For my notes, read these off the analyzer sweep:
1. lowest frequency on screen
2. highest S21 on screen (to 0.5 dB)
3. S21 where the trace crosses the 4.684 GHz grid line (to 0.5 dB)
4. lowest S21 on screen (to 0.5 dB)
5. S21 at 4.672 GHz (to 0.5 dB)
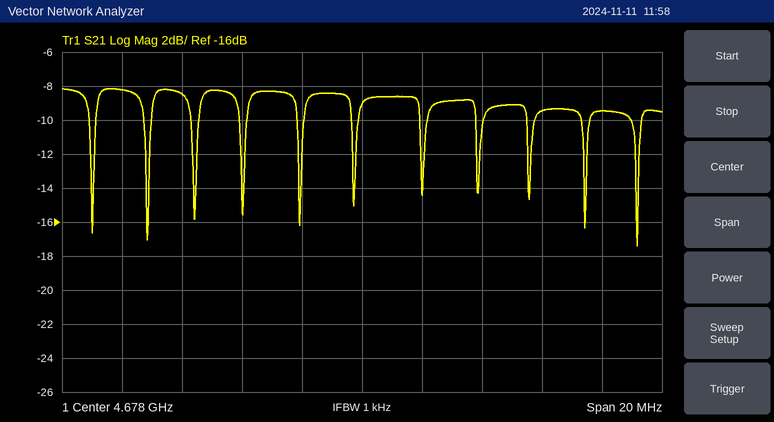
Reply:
4.668 GHz
-8.0 dB
-9.5 dB
-17.5 dB
-8.5 dB
